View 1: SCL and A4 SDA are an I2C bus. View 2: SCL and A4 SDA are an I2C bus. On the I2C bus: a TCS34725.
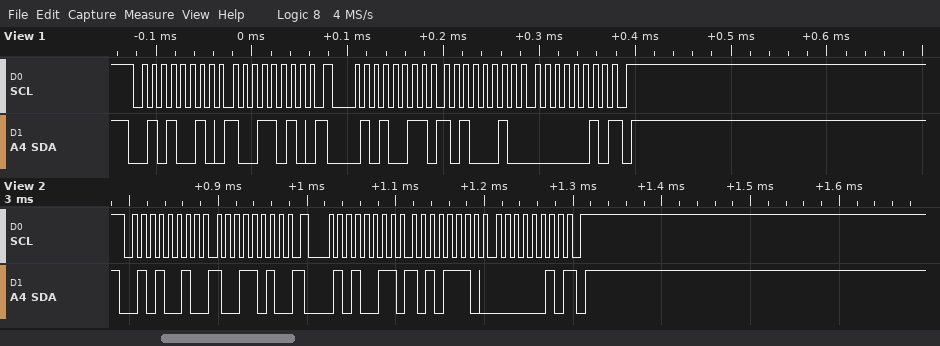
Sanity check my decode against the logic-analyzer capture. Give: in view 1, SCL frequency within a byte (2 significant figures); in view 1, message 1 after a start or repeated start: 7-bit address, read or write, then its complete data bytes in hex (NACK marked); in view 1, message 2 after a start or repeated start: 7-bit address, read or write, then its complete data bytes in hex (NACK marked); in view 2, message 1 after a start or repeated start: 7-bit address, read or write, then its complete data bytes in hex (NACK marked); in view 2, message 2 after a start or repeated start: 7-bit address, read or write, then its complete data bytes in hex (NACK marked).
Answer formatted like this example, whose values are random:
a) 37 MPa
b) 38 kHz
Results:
a) 100 kHz
b) 0x29 write: 9A
c) 0x29 read: A2 02 NACK
d) 0x29 write: 9A
e) 0x29 read: AE 02 NACK
